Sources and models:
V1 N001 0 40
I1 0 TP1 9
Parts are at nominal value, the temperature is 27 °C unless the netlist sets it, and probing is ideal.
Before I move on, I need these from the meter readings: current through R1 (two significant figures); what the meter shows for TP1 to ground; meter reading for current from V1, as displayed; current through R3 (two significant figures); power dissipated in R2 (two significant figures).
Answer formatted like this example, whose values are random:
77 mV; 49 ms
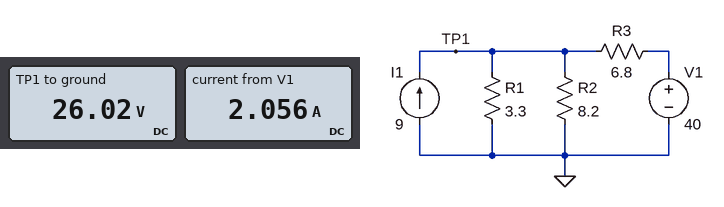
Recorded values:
7.9 A; 26.02 V; 2.056 A; 2.1 A; 83 W
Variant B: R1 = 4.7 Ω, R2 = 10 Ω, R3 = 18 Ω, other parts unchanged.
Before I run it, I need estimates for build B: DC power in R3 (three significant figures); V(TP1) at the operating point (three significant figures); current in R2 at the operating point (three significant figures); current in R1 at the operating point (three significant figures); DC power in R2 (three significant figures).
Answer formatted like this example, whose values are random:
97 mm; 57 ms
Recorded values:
5.05 W; 30.5 V; 3.05 A; 6.48 A; 92.8 W
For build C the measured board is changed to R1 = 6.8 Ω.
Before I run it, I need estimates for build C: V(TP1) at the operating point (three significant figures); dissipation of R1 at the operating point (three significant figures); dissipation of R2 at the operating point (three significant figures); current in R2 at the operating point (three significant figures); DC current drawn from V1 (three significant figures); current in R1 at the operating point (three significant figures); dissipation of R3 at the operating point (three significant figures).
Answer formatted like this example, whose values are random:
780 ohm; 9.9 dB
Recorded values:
35.8 V; 188 W; 156 W; 4.36 A; 622 mA; 5.26 A; 2.63 W
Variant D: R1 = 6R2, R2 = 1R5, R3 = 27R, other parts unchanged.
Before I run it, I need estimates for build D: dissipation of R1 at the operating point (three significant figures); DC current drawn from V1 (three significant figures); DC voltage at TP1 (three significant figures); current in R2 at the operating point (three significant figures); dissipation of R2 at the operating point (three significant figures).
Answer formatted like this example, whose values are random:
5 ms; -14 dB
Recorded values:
23.7 W; 1.03 A; 12.1 V; 8.08 A; 97.9 W
